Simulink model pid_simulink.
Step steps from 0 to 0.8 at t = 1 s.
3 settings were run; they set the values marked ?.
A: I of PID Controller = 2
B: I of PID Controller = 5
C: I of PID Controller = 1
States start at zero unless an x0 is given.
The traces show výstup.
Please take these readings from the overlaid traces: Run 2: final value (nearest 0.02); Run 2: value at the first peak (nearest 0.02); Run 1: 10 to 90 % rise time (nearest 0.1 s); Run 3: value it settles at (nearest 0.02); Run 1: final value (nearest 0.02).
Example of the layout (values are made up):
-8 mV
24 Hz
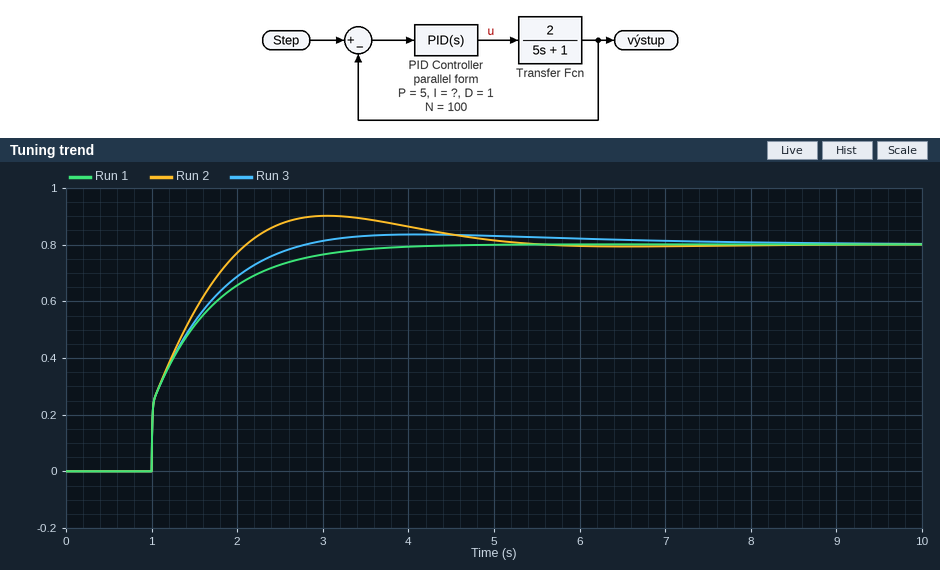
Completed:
0.80
0.90
1.4 s
0.80
0.80
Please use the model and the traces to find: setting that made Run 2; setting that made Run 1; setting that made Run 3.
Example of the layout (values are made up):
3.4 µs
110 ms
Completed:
B
C
A
